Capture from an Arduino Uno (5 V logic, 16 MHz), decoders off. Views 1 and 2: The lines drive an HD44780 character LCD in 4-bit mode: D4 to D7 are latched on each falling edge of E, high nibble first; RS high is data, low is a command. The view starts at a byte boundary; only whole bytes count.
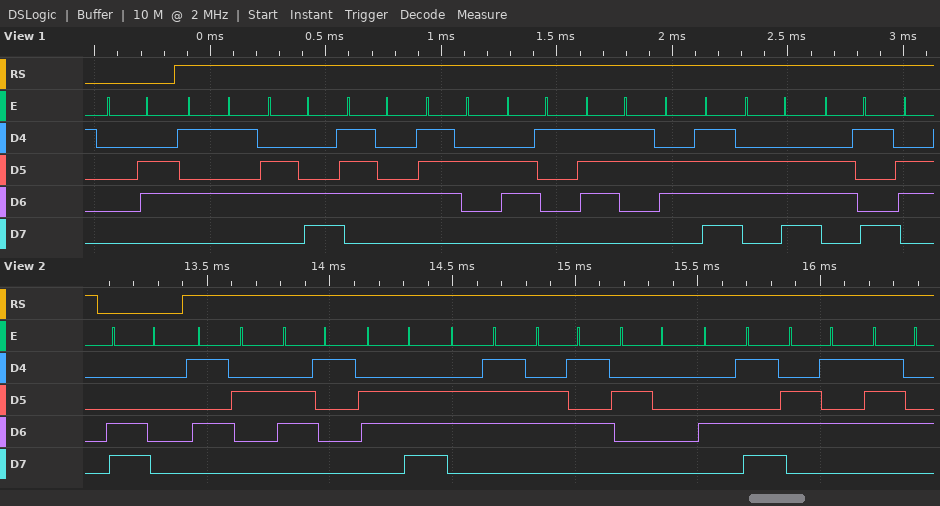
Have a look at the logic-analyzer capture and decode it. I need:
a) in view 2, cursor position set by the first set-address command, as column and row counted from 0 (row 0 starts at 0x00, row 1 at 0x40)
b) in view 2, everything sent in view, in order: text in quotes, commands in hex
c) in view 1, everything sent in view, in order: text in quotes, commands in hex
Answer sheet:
column 0, row 1
0xC0 "Range Met"
0x06 "Ultrasoni"
